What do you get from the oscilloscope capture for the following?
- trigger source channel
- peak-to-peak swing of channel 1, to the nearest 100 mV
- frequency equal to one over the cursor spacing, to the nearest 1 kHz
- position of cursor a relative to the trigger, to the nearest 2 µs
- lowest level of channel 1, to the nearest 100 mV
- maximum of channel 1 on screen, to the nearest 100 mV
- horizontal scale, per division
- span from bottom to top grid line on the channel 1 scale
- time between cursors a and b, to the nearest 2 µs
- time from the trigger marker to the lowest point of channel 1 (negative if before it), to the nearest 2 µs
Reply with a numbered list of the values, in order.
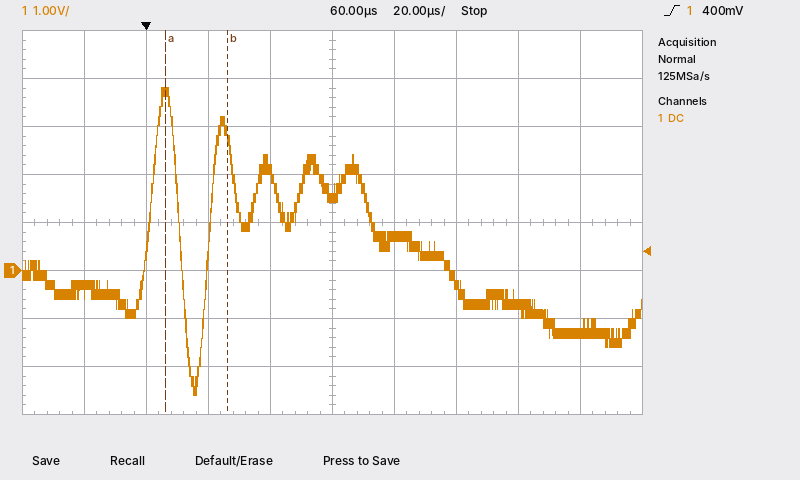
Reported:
1. channel 1
2. 6.4 V
3. 50 kHz
4. +6 µs
5. -2.6 V
6. 3.8 V
7. 20 µs
8. 8 V
9. 20 µs
10. +16 µs
